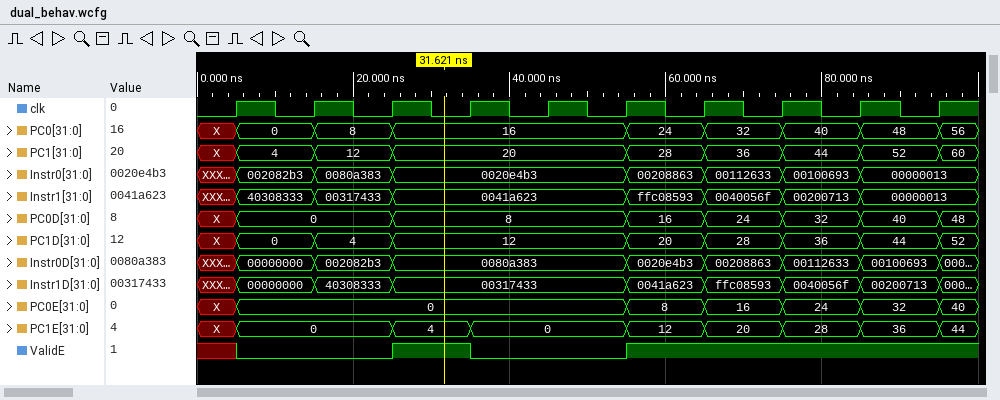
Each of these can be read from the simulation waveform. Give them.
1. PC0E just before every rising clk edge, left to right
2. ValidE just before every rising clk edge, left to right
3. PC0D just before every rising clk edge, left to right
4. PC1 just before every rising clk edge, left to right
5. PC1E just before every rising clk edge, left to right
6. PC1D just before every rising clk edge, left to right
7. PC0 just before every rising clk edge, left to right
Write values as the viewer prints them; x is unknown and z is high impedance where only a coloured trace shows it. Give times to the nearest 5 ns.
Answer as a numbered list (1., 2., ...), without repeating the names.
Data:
1. X, 0, 0, 0, 0, 0, 8, 16, 24, 32
2. x 0 0 1 0 0 1 1 1 1
3. X, 0, 0, 8, 8, 8, 16, 24, 32, 40
4. X, 4, 12, 20, 20, 20, 28, 36, 44, 52
5. X, 0, 0, 4, 0, 0, 12, 20, 28, 36
6. X, 0, 4, 12, 12, 12, 20, 28, 36, 44
7. X, 0, 8, 16, 16, 16, 24, 32, 40, 48
